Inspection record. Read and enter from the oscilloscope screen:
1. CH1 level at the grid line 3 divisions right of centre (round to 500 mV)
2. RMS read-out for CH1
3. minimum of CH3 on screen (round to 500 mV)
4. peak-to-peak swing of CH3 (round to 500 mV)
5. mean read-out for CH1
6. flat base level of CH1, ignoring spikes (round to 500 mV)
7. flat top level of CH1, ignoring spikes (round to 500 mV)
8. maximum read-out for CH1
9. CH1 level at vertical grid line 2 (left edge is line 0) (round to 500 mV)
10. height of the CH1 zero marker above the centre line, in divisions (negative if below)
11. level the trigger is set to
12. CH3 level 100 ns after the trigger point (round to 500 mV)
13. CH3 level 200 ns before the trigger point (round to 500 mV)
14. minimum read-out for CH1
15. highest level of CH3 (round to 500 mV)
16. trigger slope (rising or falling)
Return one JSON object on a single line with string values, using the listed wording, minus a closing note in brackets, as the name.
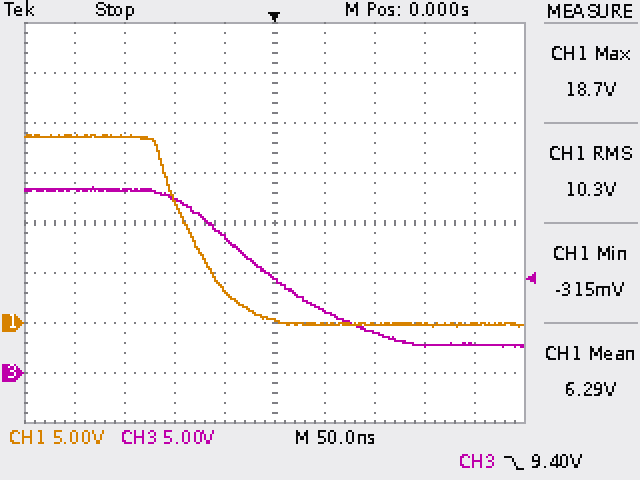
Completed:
{"CH1 level at the grid line 3 divisions right of centre": "0.0 V", "RMS read-out for CH1": "10.3 V", "minimum of CH3 on screen": "2.5 V", "peak-to-peak swing of CH3": "16.0 V", "mean read-out for CH1": "6.29 V", "flat base level of CH1, ignoring spikes": "0.0 V", "flat top level of CH1, ignoring spikes": "18.5 V", "maximum read-out for CH1": "18.7 V", "CH1 level at vertical grid line 2 (left edge is line 0)": "18.5 V", "height of the CH1 zero marker above the centre line, in divisions": "-2.0 div", "level the trigger is set to": "9.40 V", "CH3 level 100 ns after the trigger point": "4.0 V", "CH3 level 200 ns before the trigger point": "18.5 V", "minimum read-out for CH1": "-315 mV", "highest level of CH3": "18.5 V", "trigger slope": "falling"}
